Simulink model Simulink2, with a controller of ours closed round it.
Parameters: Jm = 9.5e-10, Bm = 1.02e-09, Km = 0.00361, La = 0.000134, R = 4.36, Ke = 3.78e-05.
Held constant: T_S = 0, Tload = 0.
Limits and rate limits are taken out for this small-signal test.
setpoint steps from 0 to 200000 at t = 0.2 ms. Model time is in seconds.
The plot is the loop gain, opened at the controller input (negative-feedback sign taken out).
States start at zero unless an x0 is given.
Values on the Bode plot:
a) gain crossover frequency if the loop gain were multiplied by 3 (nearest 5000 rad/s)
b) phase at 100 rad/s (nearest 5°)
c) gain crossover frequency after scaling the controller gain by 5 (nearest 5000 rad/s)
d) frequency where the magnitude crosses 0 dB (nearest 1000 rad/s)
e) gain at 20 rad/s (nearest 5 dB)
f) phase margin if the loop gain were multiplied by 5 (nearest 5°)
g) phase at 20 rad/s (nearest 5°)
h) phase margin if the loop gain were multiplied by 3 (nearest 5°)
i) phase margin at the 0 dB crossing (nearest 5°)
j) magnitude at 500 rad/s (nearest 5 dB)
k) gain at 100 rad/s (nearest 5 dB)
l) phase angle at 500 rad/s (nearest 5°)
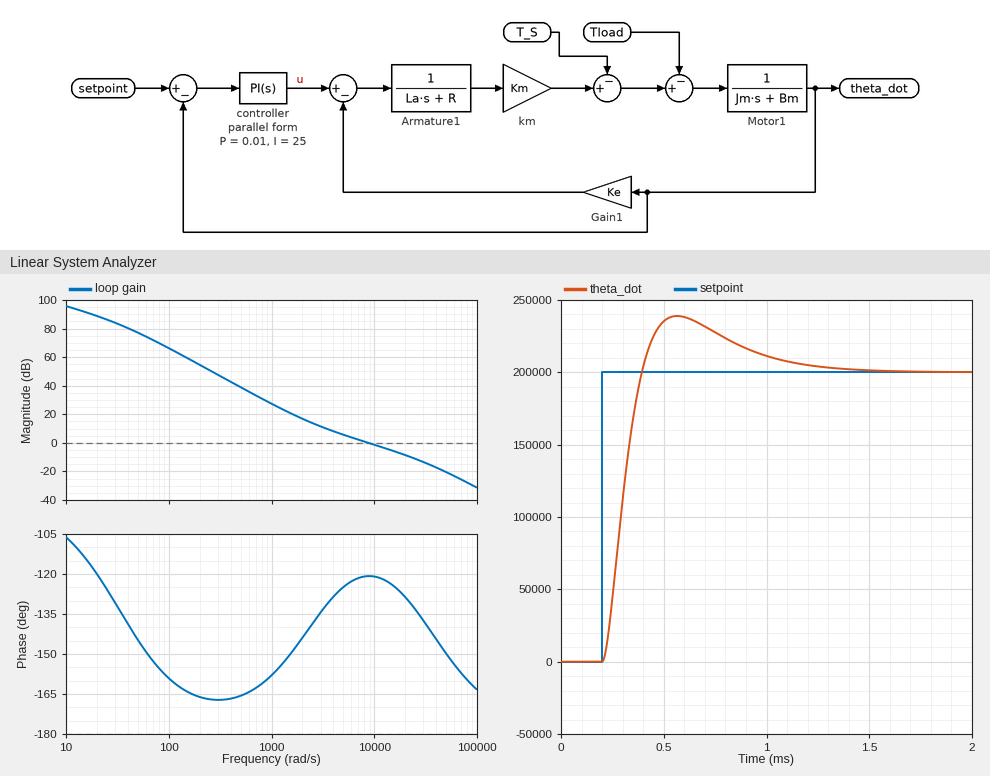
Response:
20000 rad/s
-160°
30000 rad/s
9000 rad/s
90 dB
40°
-120°
50°
60°
40 dB
65 dB
-165°
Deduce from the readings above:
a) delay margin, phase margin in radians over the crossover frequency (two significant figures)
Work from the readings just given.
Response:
0.00012 s
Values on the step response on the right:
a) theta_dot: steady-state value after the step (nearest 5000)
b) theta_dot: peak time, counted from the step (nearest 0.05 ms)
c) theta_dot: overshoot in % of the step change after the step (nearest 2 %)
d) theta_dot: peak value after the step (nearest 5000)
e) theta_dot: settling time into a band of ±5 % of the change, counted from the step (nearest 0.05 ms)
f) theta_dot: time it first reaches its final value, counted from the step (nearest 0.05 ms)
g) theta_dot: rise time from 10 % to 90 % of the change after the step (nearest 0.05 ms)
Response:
200000
0.35 ms
20 %
240000
0.85 ms
0.20 ms
0.15 ms
